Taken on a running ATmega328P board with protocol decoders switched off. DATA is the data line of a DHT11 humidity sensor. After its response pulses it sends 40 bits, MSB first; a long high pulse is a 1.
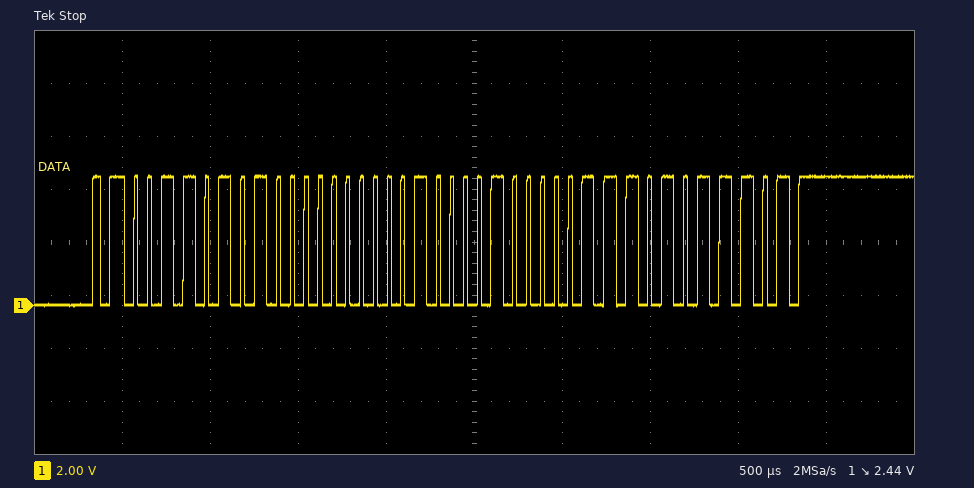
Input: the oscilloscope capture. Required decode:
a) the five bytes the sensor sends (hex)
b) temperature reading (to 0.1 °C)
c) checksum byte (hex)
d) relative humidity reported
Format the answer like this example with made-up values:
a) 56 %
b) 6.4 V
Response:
a) 35 00 21 07 5D
b) 33.7 °C
c) 0x5D
d) 53 %
